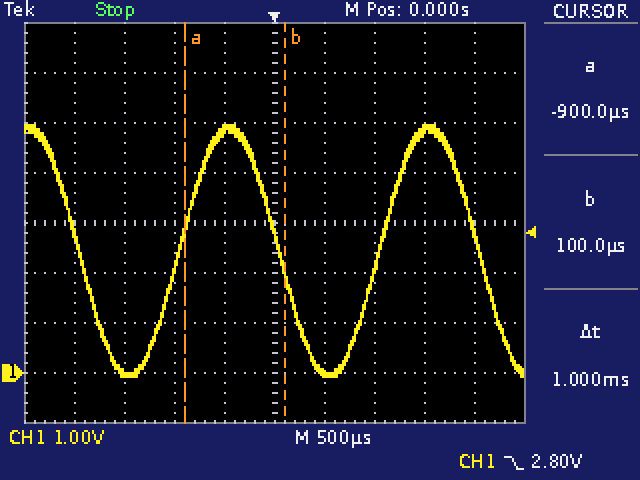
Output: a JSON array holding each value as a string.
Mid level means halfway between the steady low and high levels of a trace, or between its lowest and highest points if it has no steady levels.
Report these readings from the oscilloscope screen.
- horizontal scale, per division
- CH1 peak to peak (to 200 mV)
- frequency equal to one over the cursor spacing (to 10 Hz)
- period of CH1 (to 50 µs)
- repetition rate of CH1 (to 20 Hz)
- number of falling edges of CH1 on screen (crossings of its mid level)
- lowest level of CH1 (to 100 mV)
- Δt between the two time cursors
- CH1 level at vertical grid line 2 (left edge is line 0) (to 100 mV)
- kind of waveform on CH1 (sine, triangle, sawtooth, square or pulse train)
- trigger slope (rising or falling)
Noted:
["500 µs", "5.0 V", "1.00 kHz", "2.00 ms", "500 Hz", "3", "-100 mV", "1 ms", "0.0 V", "sine", "falling"]
